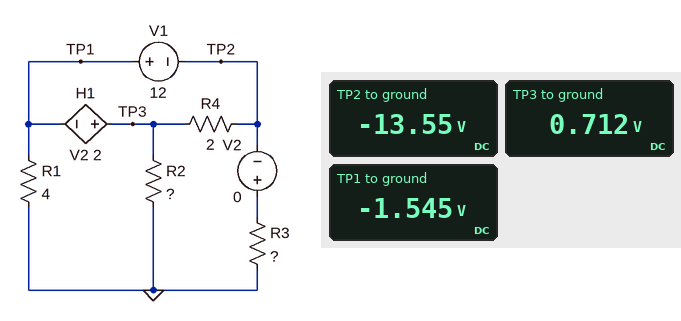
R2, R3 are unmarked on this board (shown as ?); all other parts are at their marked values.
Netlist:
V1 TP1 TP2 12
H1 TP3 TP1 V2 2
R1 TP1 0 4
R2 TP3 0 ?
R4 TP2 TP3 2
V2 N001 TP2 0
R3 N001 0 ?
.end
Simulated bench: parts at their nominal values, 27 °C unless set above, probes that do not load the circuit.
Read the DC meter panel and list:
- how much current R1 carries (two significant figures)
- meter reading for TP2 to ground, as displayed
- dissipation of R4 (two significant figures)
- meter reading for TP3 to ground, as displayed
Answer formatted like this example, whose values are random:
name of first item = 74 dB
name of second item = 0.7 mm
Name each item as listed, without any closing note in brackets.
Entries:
how much current R1 carries = 390 mA
meter reading for TP2 to ground, as displayed = -13.55 V
dissipation of R4 = 100 W
meter reading for TP3 to ground, as displayed = 0.712 V
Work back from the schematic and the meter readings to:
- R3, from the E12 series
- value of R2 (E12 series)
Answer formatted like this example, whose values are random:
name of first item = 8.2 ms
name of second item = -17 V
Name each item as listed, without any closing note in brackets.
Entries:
R3, from the E12 series = 12 Ω
value of R2 = 0.47 Ω
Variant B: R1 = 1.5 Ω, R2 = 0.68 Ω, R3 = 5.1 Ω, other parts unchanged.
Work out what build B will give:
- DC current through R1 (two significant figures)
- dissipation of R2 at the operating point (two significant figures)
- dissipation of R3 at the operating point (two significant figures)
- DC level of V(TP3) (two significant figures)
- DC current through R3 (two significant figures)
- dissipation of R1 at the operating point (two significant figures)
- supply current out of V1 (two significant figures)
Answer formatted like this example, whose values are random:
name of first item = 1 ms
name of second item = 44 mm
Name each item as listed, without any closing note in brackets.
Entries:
DC current through R1 = 1.7 A
dissipation of R2 at the operating point = 14 W
dissipation of R3 at the operating point = 42 W
DC level of V(TP3) = 3.1 V
DC current through R3 = 2.9 A
dissipation of R1 at the operating point = 4.5 W
supply current out of V1 = 12 A
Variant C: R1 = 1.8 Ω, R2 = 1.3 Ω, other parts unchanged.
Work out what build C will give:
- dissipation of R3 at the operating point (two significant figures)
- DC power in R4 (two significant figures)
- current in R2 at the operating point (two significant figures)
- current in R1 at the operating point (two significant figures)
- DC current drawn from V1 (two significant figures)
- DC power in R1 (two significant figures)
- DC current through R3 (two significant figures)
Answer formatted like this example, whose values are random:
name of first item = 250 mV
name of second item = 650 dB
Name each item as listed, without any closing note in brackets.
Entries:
dissipation of R3 at the operating point = 13 W
DC power in R4 = 99 W
current in R2 at the operating point = 1.3 A
current in R1 at the operating point = 230 mA
DC current drawn from V1 = 8.1 A
DC power in R1 = 98 mW
DC current through R3 = 1.0 A
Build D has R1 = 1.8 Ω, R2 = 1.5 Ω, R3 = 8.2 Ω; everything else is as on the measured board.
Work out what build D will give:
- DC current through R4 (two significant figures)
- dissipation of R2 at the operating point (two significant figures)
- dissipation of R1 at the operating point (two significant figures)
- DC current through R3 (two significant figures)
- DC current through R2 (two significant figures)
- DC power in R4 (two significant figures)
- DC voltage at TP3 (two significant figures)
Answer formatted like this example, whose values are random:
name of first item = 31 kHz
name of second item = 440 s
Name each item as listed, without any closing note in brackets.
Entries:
DC current through R4 = 7.5 A
dissipation of R2 at the operating point = 4.6 W
dissipation of R1 at the operating point = 95 mW
DC current through R3 = 1.5 A
DC current through R2 = 1.7 A
DC power in R4 = 110 W
DC voltage at TP3 = 2.6 V
